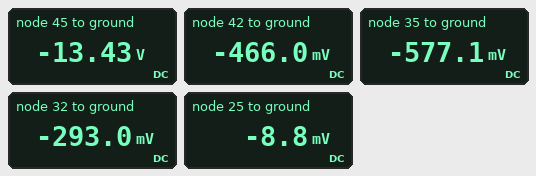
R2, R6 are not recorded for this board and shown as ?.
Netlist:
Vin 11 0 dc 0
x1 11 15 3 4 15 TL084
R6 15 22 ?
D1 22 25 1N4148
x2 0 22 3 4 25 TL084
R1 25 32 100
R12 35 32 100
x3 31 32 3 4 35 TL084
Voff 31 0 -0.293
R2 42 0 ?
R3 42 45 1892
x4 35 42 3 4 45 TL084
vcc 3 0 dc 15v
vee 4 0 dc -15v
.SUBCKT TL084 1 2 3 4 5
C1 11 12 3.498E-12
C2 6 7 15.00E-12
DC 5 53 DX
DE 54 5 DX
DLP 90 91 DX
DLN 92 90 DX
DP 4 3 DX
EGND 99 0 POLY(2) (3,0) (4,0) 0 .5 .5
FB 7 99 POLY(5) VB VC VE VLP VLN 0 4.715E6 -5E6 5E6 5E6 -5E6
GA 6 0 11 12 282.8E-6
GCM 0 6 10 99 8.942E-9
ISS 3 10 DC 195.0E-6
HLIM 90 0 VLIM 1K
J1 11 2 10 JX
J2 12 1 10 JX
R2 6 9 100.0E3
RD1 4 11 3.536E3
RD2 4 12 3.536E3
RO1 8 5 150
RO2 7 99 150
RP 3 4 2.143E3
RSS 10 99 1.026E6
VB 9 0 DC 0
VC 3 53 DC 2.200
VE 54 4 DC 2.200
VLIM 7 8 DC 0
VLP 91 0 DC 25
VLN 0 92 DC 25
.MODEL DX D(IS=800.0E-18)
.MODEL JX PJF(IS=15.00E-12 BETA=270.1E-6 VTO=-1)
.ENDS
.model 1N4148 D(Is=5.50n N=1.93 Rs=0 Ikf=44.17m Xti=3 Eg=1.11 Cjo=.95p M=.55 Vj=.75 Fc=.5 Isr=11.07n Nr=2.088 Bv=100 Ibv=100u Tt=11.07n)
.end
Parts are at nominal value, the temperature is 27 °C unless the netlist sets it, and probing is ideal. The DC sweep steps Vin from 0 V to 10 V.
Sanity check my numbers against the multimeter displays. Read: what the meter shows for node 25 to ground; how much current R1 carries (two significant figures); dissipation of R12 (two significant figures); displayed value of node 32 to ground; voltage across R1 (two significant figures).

-8.8 mV
2.8 mA
810 µW
-293.0 mV
280 mV
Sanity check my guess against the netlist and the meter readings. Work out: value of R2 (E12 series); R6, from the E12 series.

68 Ω
1.2 kΩ
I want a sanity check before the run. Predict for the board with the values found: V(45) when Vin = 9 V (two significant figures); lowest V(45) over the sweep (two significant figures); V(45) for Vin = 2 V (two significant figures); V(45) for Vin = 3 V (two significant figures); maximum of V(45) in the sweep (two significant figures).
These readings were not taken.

3.8 V
-13 V
1.2 V
1.9 V
4.0 V
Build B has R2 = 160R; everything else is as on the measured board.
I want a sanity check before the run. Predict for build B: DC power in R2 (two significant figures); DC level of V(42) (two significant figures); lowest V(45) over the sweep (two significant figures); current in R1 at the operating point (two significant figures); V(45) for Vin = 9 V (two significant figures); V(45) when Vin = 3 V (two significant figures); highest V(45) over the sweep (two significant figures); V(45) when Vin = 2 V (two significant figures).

2.1 mW
-580 mV
-7.4 V
2.8 mA
1.7 V
830 mV
1.8 V
520 mV
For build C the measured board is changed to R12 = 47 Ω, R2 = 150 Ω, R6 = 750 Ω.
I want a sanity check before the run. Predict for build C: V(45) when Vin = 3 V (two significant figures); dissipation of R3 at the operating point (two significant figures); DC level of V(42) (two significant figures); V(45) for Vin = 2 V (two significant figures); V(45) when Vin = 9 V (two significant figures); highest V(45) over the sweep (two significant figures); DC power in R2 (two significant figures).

-1.5 V
15 mW
-420 mV
-1.7 V
-1.1 V
-1.0 V
1.2 mW
